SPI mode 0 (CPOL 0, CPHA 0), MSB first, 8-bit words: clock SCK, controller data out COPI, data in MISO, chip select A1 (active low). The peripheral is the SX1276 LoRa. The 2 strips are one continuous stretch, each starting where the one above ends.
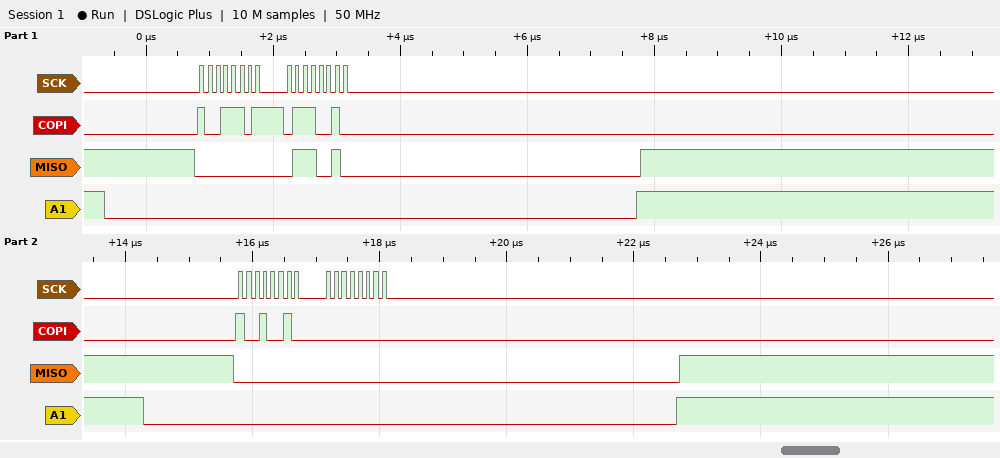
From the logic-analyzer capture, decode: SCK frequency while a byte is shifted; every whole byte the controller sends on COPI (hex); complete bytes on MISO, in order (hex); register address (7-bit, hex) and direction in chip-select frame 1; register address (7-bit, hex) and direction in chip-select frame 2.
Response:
8 MHz
0x9D 0x72 0x92 0x00
0x00 0x72 0x00 0x00
0x1D write
0x12 write
